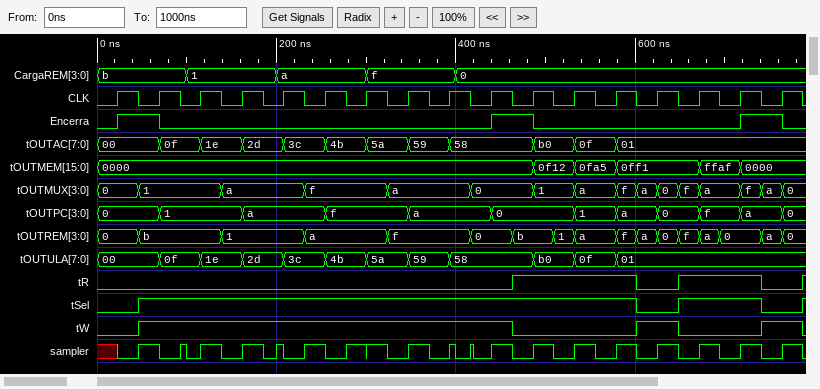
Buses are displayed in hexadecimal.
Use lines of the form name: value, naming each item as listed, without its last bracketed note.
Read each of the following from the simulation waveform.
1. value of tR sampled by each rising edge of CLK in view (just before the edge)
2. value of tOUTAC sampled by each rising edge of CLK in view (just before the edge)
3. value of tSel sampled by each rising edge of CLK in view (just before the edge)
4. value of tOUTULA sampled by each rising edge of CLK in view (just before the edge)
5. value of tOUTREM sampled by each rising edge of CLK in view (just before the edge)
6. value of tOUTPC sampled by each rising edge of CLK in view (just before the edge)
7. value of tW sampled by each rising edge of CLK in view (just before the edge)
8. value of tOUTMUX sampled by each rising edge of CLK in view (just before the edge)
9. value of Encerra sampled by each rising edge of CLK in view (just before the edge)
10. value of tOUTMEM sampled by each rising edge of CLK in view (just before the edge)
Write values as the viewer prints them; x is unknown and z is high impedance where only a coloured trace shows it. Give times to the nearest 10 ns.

value of tR sampled by each rising edge of CLK in view: 0 0 0 0 0 0 0 0 0 0 1 1 1 0 1 1 0
value of tOUTAC sampled by each rising edge of CLK in view: 00, 00, 0f, 1e, 2d, 3c, 4b, 5a, 59, 58, 58, b0, 0f, 01, 01, 01, 01
value of tSel sampled by each rising edge of CLK in view: 0 1 1 1 1 1 1 1 1 1 1 1 1 0 1 1 0
value of tOUTULA sampled by each rising edge of CLK in view: 00, 00, 0f, 1e, 2d, 3c, 4b, 5a, 59, 58, 58, b0, 0f, 01, 01, 01, 01
value of tOUTREM sampled by each rising edge of CLK in view: 0, b, b, 1, 1, a, a, f, f, 0, b, 1, a, a, f, 0, a
value of tOUTPC sampled by each rising edge of CLK in view: 0, 0, 1, 1, a, a, f, f, a, a, 0, 0, 1, a, 0, f, a
value of tW sampled by each rising edge of CLK in view: 0 1 1 1 1 1 1 1 1 1 0 0 0 1 0 0 1
value of tOUTMUX sampled by each rising edge of CLK in view: 0, 1, 1, a, a, f, f, a, a, 0, 0, 1, a, a, f, a, a
value of Encerra sampled by each rising edge of CLK in view: 0 1 0 0 0 0 0 0 0 0 1 0 0 0 0 0 1
value of tOUTMEM sampled by each rising edge of CLK in view: 0000, 0000, 0000, 0000, 0000, 0000, 0000, 0000, 0000, 0000, 0000, 0f12, 0fa5, 0ff1, 0ff1, ffaf, 0000
